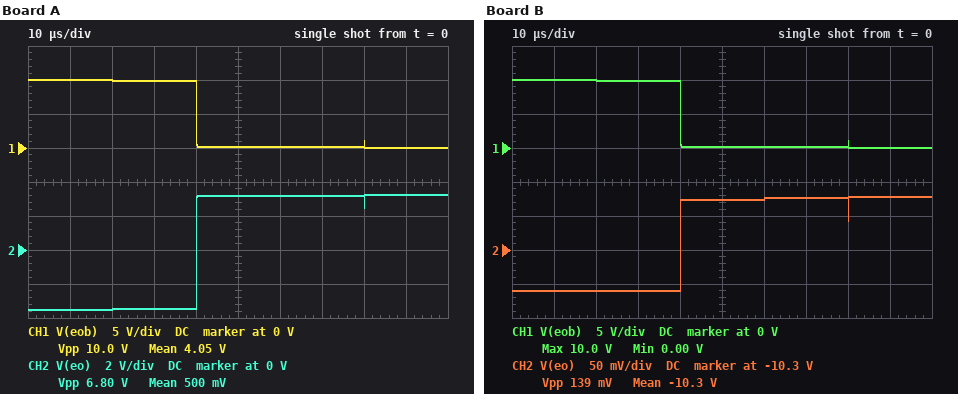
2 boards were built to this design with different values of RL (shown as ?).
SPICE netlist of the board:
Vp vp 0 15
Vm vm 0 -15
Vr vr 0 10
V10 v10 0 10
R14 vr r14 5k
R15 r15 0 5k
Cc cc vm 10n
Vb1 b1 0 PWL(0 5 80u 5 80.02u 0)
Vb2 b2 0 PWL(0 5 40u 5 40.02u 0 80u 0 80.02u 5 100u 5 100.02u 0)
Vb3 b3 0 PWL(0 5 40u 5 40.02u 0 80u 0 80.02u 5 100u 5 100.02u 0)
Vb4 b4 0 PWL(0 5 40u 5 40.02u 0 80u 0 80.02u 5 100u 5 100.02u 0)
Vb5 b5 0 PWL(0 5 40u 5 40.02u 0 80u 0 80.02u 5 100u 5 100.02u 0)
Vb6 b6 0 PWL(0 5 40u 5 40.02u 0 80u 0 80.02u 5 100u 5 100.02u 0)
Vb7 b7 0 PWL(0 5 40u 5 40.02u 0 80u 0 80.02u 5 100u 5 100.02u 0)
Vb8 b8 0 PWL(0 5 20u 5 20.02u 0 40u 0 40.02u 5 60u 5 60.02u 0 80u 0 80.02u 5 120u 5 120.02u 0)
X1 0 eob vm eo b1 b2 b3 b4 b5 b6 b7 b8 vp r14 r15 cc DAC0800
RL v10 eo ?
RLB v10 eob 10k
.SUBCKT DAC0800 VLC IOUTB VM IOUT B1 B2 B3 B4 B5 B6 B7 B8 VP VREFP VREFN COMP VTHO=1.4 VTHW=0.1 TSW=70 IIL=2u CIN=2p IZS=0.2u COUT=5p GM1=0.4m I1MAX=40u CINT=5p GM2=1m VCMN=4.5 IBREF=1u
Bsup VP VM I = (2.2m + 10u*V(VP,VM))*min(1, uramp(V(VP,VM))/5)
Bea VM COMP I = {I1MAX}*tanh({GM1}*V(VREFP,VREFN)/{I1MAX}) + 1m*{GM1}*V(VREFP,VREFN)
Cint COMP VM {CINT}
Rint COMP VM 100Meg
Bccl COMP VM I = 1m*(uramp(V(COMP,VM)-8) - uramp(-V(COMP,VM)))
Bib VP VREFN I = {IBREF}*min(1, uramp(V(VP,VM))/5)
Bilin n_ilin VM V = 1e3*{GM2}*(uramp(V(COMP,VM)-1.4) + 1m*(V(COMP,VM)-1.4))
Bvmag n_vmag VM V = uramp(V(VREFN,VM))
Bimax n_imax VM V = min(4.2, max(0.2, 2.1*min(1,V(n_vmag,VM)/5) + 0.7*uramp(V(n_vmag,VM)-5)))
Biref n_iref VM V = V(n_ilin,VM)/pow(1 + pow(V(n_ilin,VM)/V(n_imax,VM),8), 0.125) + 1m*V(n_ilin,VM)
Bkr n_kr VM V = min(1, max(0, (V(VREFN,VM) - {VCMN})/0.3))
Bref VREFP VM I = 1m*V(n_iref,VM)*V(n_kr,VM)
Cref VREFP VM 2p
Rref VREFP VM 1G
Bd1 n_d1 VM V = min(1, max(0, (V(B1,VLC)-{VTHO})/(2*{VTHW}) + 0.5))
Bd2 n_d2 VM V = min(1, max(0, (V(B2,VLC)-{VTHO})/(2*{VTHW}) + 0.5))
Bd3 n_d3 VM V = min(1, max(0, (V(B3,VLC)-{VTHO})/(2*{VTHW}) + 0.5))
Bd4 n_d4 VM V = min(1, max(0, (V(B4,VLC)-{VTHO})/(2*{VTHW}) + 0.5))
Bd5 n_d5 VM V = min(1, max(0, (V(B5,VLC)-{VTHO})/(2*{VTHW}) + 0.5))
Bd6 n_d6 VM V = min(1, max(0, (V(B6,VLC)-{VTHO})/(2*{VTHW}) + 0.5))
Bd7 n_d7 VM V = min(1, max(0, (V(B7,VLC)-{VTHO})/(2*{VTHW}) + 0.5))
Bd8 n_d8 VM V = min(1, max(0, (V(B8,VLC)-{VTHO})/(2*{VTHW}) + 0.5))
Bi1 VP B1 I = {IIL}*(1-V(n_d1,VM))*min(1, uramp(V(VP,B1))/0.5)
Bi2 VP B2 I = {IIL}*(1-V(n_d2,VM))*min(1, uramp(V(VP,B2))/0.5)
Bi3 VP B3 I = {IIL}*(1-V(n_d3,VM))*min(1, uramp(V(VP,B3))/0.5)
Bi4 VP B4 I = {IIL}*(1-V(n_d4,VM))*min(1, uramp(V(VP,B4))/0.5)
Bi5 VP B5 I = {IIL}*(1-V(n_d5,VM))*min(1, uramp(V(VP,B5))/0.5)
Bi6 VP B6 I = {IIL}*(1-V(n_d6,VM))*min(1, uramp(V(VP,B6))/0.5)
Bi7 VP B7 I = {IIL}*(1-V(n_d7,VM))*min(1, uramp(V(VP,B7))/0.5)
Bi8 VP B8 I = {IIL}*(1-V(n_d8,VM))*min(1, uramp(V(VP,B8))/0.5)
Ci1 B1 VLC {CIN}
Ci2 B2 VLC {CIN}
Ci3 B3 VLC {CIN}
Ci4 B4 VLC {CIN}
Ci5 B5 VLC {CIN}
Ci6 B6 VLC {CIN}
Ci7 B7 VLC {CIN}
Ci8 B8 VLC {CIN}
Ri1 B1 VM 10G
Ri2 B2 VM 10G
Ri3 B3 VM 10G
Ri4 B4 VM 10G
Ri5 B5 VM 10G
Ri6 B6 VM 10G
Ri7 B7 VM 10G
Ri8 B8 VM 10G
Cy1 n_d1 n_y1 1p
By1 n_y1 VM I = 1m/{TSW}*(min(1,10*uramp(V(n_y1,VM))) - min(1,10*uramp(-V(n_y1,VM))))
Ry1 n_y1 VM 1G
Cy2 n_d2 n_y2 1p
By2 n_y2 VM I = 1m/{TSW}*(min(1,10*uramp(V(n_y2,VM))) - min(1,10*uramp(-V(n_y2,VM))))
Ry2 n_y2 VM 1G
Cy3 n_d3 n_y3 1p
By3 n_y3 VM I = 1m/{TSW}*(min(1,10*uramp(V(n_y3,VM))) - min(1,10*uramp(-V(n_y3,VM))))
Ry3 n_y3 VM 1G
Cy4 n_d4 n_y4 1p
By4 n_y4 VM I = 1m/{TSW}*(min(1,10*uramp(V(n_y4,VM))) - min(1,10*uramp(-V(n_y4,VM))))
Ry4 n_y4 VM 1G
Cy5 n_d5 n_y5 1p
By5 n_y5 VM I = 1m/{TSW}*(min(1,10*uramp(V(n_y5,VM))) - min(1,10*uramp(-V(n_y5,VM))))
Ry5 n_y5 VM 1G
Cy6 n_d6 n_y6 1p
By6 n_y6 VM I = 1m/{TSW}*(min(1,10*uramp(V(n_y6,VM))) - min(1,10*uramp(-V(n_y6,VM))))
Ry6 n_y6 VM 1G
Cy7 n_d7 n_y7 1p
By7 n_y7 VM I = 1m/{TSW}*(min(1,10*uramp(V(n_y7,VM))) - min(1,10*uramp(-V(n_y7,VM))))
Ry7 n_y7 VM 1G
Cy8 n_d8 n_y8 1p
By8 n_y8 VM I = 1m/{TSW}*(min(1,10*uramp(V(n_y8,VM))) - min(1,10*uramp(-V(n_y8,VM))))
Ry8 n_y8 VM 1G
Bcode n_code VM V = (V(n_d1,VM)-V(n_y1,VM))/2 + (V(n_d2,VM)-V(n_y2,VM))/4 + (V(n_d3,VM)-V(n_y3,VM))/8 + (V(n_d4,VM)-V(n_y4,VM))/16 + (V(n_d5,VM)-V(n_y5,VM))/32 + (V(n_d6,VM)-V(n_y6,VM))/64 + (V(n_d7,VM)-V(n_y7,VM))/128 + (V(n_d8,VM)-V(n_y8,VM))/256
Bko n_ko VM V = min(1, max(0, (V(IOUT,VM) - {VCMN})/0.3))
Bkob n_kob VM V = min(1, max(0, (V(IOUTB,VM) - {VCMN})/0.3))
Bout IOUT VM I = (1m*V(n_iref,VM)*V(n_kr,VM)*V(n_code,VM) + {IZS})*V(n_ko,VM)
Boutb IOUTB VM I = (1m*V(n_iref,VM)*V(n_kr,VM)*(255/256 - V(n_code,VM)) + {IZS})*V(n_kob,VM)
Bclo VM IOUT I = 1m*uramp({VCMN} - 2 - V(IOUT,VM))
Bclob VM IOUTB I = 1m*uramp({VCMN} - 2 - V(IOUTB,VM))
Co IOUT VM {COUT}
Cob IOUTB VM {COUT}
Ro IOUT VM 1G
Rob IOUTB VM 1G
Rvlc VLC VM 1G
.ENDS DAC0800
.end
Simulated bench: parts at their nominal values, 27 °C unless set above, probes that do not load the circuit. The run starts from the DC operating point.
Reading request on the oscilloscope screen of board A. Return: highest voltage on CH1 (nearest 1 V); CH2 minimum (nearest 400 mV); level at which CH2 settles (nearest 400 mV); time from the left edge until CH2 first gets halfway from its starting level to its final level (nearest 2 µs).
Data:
10 V
-3.6 V
3.2 V
40 µs
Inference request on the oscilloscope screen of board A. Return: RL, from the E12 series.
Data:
6.8 kΩ
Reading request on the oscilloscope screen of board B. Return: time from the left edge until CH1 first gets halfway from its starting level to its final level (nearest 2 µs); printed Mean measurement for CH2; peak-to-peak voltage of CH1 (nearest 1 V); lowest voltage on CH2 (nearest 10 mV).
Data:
40 µs
-10.3 V
10 V
-10.36 V
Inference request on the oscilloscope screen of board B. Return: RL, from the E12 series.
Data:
22 kΩ
